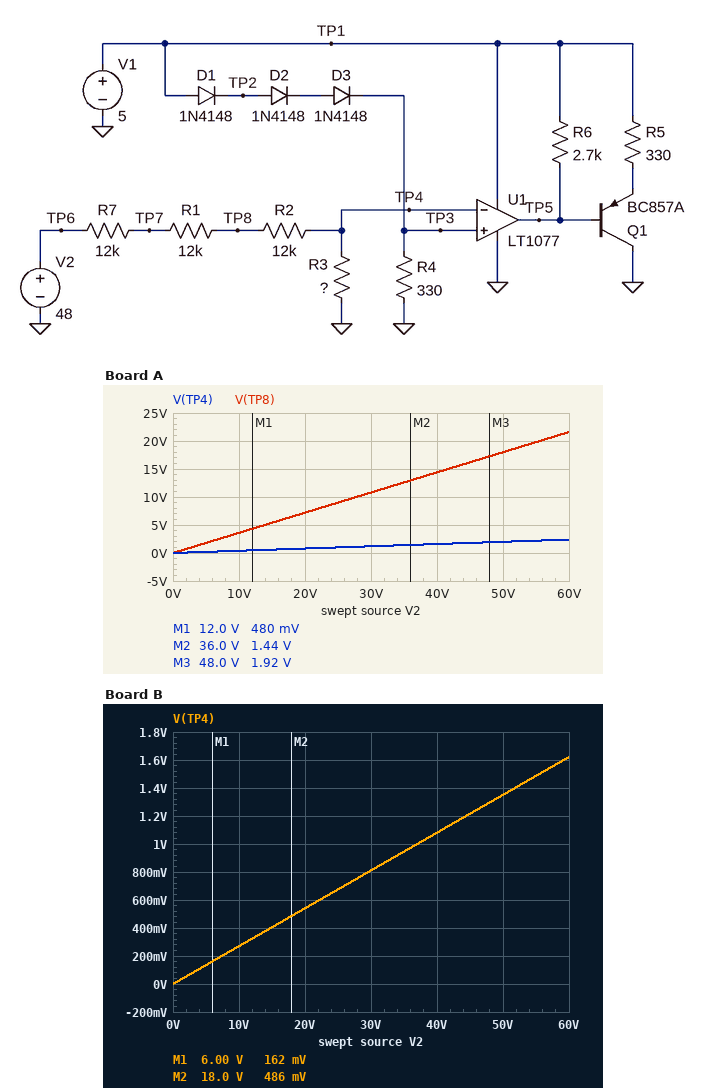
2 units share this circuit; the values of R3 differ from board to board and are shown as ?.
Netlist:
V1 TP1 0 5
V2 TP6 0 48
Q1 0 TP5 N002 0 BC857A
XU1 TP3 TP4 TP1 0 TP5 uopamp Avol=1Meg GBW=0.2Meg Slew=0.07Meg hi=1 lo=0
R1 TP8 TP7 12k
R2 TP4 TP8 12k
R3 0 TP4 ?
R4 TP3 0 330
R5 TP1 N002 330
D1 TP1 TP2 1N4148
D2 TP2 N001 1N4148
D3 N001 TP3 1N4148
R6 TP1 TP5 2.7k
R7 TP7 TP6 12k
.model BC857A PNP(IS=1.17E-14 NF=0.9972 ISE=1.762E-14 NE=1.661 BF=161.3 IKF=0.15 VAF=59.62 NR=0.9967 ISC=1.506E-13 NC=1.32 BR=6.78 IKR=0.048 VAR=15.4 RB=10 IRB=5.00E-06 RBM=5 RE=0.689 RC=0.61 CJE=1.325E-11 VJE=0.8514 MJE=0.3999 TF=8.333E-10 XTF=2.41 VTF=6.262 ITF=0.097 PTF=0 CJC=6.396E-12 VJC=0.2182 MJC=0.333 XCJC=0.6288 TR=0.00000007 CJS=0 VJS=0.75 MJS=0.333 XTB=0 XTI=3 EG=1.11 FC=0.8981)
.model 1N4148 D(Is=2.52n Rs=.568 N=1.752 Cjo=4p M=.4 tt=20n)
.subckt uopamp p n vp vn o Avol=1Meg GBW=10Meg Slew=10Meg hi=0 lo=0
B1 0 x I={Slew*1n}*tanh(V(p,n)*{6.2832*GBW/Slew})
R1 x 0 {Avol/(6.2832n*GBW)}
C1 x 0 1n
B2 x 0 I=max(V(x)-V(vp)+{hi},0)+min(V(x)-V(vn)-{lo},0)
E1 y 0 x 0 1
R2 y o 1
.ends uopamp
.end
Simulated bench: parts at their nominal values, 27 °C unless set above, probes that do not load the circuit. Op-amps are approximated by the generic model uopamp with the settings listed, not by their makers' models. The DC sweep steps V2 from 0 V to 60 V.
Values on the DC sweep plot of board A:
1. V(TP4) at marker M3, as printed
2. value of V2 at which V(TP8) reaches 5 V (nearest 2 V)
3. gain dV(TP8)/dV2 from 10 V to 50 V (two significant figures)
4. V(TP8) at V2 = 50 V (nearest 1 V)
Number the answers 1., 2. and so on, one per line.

1. 1.92 V
2. 14 V
3. 0.36 V/V
4. 18 V
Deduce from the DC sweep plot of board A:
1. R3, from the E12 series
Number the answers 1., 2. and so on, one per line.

1. 1.5 kΩ
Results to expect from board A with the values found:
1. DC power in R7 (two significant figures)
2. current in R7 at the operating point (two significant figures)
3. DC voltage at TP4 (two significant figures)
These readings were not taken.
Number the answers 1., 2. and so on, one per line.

1. 20 mW
2. 1.3 mA
3. 1.9 V
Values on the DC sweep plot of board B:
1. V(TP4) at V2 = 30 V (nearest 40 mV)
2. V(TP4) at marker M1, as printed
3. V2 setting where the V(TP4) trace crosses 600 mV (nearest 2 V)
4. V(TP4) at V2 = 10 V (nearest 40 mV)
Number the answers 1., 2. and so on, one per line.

1. 800 mV
2. 162 mV
3. 22 V
4. 280 mV
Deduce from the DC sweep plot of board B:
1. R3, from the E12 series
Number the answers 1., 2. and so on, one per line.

1. 1 kΩ
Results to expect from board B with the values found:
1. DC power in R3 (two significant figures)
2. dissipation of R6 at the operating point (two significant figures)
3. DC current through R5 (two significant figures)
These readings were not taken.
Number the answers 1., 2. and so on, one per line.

1. 1.7 mW
2. 370 µW
3. 1.1 mA
